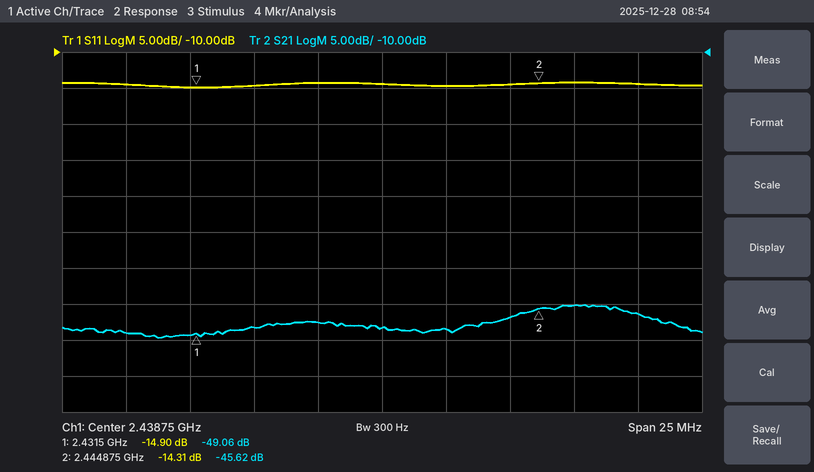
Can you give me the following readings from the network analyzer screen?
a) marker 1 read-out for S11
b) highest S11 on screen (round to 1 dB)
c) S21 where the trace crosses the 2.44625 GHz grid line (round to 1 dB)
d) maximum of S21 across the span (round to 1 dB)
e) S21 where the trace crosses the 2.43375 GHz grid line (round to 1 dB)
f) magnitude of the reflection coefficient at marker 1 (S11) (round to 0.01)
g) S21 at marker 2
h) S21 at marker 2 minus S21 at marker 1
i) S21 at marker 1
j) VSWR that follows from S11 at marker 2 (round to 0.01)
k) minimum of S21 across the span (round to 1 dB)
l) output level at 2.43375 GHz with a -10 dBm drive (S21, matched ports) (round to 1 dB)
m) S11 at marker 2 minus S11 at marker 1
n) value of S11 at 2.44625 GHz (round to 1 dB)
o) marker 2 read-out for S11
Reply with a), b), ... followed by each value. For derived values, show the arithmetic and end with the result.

a) -14.90 dB
b) -14 dB
c) -45 dB
d) -45 dB
e) -48 dB
f) 10^(-14.9/20) ≈ 0.18
g) -45.62 dB
h) -45.62 − (-49.06) = 3.44 dB
i) -49.06 dB
j) (1 + 0.1925)/(1 − 0.1925) ≈ 1.48
k) -50 dB
l) -10 dBm + (-48 dB) = -58 dBm
m) -14.31 − (-14.9) = 0.59 dB
n) -14 dB
o) -14.31 dB
